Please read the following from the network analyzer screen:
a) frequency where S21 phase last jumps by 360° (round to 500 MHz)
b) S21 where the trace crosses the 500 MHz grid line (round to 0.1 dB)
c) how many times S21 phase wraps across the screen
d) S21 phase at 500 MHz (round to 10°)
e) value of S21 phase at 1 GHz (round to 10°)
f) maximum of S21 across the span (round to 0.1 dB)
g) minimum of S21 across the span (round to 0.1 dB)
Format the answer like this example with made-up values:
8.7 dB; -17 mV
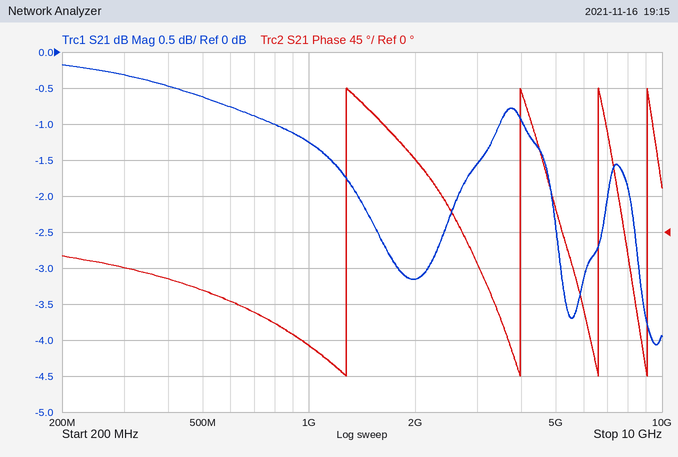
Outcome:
9.0 GHz; -0.6 dB; 4; -70°; -140°; -0.2 dB; -4.1 dB
